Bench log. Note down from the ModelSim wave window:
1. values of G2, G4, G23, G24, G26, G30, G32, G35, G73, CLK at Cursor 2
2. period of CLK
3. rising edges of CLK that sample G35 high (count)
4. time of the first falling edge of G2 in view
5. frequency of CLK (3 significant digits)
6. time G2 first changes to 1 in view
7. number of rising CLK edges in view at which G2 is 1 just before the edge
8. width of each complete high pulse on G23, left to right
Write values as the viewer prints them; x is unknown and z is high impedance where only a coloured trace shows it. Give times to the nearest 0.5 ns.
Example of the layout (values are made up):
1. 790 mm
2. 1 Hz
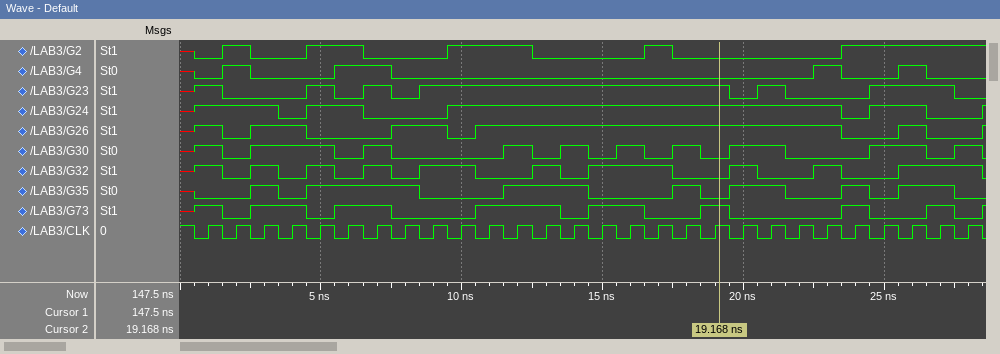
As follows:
1. G2=0, G4=0, G23=1, G24=1, G26=1, G30=0, G32=0, G35=0, G73=1, CLK=1
2. 1 ns
3. 14
4. 2.5 ns
5. 1.00 GHz
6. 1.5 ns
7. 12
8. 1 ns, 1 ns, 11 ns, 1 ns, 3 ns
